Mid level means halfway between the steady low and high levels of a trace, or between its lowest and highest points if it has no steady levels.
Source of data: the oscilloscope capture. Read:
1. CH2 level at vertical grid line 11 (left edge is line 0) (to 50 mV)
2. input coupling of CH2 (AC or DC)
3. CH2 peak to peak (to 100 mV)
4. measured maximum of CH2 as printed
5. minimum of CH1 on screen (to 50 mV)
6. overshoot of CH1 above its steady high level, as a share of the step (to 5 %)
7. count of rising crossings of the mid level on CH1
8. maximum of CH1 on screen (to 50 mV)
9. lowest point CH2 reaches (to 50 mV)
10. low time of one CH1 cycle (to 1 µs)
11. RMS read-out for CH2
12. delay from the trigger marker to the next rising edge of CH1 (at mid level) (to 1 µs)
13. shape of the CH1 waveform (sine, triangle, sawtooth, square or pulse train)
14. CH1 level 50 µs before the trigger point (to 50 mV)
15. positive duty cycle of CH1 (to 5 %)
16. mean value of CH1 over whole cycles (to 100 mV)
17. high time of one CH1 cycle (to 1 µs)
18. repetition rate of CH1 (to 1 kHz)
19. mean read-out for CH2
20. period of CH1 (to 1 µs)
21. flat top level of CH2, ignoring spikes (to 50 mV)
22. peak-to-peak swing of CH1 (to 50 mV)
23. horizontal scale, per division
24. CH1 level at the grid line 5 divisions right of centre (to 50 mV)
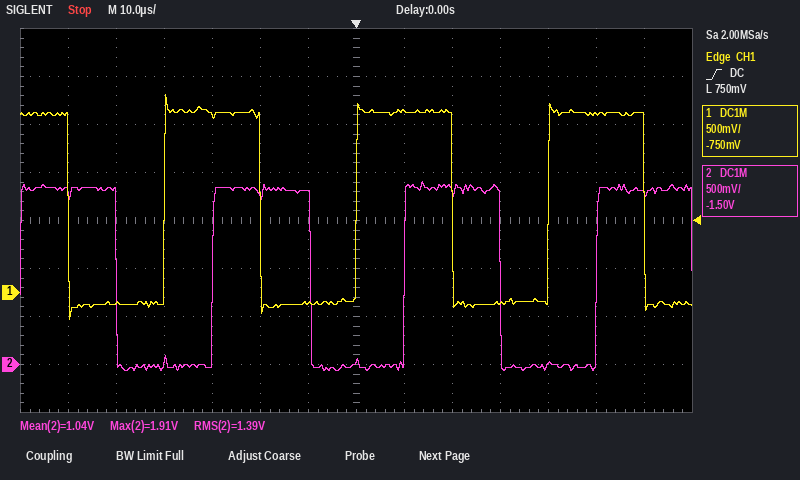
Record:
0 mV
DC
2.00 V
1.91 V
-300 mV
10 %
3
2.05 V
-50 mV
20 µs
1.39 V
40 µs
square
-100 mV
50 %
900 mV
20 µs
25 kHz
1.04 V
40 µs
1.85 V
2.35 V
10 µs
1.85 V
